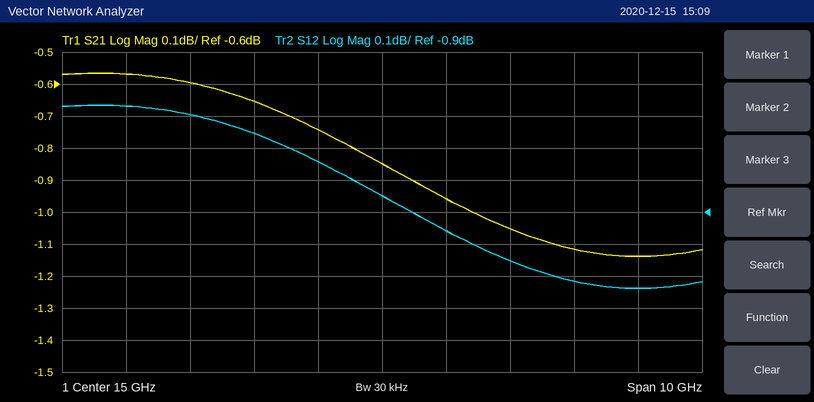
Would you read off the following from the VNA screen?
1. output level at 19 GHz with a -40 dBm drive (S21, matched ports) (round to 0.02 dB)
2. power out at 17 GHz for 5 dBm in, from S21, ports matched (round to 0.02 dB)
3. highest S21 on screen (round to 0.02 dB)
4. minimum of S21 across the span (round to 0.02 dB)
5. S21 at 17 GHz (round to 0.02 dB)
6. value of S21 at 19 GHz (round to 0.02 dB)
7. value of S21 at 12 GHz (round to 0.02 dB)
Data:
-41.14 dBm
3.94 dBm
-0.56 dB
-1.14 dB
-1.06 dB
-1.14 dB
-0.60 dB
